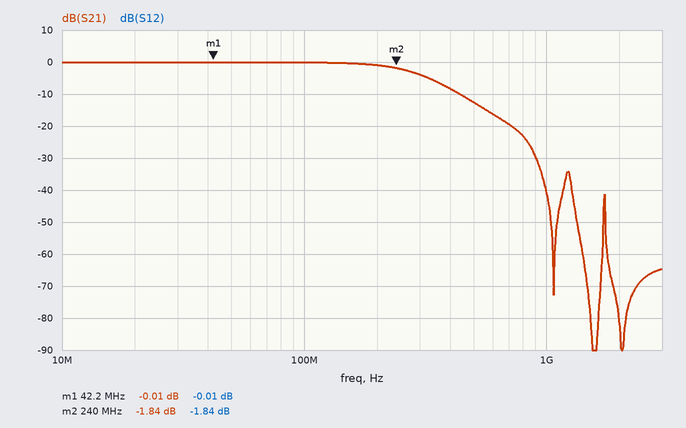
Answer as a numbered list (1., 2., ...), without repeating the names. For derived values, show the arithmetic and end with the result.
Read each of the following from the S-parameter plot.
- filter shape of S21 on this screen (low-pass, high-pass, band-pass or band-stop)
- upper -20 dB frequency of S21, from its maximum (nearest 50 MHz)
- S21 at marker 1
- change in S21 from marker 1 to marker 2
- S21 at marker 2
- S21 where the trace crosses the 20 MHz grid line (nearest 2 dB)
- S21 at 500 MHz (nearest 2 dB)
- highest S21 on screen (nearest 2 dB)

1. low-pass
2. 700 MHz
3. -0.01 dB
4. -1.84 − (-0.01) = -1.83 dB
5. -1.84 dB
6. 0 dB
7. -12 dB
8. 0 dB
